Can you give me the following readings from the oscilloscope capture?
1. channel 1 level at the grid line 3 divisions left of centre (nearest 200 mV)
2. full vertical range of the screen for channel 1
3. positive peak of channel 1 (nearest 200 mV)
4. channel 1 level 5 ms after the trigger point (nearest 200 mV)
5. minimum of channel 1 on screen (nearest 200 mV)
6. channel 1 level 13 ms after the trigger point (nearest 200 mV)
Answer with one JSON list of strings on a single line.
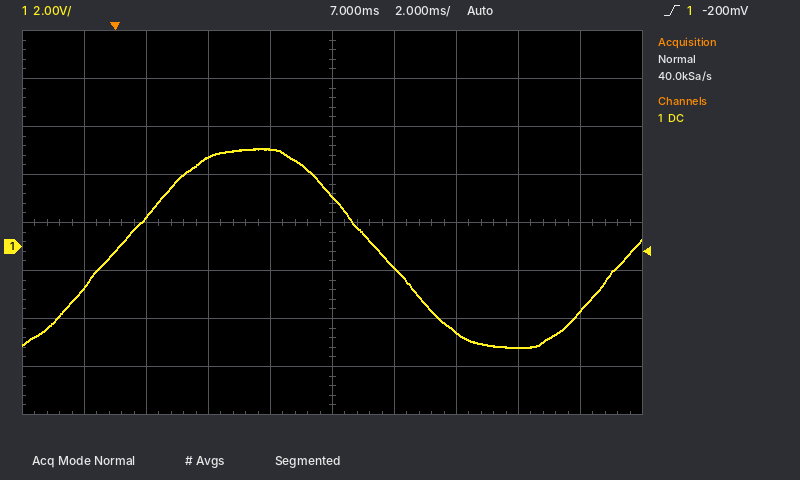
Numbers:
["1.2 V", "16 V", "4.0 V", "4.0 V", "-4.2 V", "-4.2 V"]
